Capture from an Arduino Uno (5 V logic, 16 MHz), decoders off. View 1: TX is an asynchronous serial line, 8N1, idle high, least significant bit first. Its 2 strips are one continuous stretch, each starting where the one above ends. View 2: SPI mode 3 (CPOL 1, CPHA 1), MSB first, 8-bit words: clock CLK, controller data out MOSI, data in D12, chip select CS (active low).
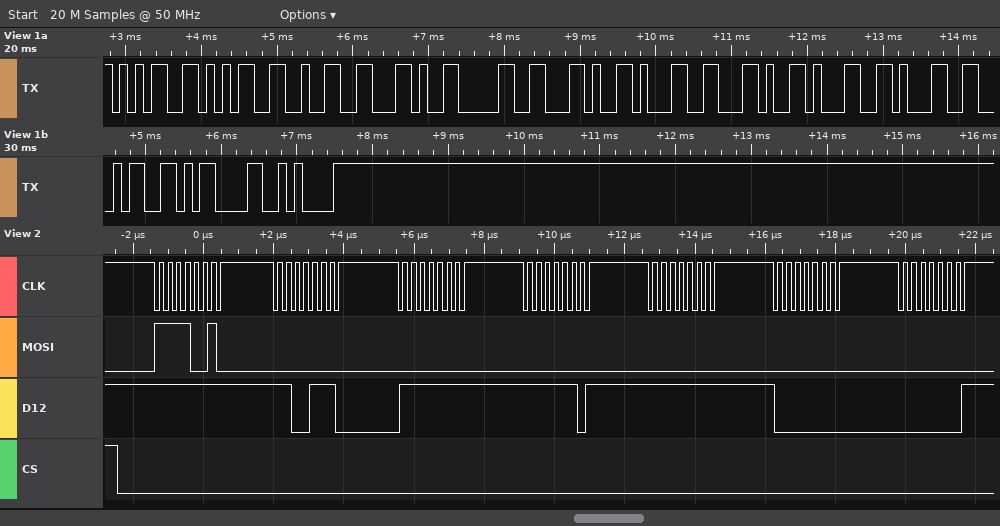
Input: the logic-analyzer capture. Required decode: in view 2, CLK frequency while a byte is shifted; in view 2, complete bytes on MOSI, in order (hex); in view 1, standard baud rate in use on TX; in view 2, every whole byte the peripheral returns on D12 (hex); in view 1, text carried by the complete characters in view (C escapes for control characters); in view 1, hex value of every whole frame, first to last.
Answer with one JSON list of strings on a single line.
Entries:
["4 MHz", "F2 00 00 00 00 00 00", "9600 baud", "FF CE FF FD FF 00 01", "\"552,0,1,114\\r\\n\"", "0x35 0x35 0x32 0x2C 0x30 0x2C 0x31 0x2C 0x31 0x31 0x34 0x0D 0x0A"]
